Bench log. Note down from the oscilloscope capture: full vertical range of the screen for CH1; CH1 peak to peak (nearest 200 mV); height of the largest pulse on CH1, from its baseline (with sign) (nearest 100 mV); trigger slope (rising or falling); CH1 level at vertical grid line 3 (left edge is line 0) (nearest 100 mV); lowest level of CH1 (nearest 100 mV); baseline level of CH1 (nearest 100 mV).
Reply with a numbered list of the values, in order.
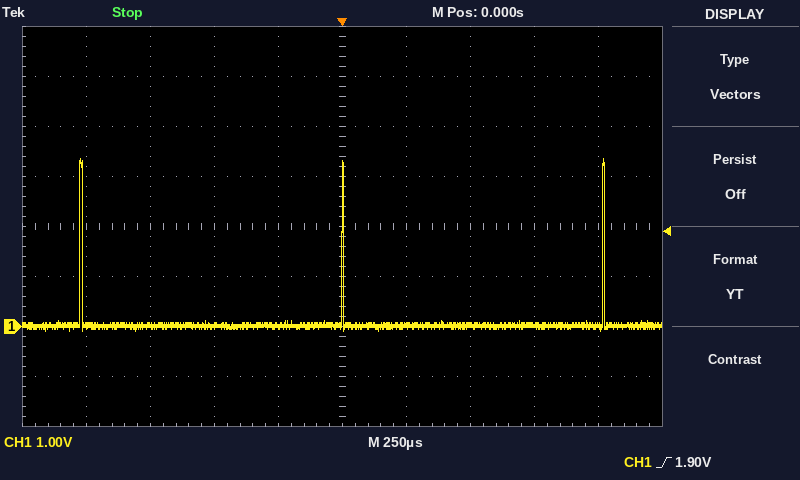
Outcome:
1. 8 V
2. 3.4 V
3. +3.3 V
4. rising
5. 0.0 V
6. -100 mV
7. 0.0 V
